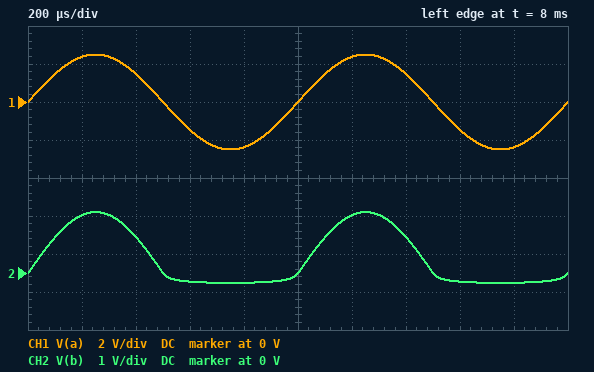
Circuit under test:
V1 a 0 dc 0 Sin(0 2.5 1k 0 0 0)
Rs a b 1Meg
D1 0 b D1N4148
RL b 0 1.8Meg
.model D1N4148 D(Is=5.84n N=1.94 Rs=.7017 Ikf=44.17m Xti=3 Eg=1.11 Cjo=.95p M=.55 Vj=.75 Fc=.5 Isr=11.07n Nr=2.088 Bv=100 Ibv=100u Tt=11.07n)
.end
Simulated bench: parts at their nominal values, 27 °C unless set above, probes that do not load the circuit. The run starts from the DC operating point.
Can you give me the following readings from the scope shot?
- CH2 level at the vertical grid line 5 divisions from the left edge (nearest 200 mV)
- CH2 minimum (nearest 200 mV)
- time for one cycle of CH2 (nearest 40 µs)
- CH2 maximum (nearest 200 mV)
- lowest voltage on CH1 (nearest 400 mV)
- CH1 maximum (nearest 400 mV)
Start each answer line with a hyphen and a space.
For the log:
- 0 V
- -200 mV
- 1.00 ms
- 1.6 V
- -2.4 V
- 2.4 V
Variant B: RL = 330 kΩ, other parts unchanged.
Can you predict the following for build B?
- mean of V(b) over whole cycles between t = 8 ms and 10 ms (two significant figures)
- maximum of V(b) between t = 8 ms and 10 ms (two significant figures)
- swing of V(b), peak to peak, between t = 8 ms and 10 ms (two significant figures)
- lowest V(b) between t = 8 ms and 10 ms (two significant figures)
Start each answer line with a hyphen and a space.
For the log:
- 100 mV
- 620 mV
- 860 mV
- -240 mV
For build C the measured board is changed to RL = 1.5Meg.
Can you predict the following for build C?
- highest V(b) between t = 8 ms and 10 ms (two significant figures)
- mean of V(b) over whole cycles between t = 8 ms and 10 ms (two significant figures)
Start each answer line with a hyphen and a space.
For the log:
- 1.5 V
- 370 mV
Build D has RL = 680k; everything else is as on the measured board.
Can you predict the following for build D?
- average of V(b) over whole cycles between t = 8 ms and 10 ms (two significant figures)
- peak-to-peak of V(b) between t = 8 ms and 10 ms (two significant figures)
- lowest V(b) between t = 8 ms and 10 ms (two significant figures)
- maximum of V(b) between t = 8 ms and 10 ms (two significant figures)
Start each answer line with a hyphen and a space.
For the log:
- 220 mV
- 1.3 V
- -250 mV
- 1.0 V
